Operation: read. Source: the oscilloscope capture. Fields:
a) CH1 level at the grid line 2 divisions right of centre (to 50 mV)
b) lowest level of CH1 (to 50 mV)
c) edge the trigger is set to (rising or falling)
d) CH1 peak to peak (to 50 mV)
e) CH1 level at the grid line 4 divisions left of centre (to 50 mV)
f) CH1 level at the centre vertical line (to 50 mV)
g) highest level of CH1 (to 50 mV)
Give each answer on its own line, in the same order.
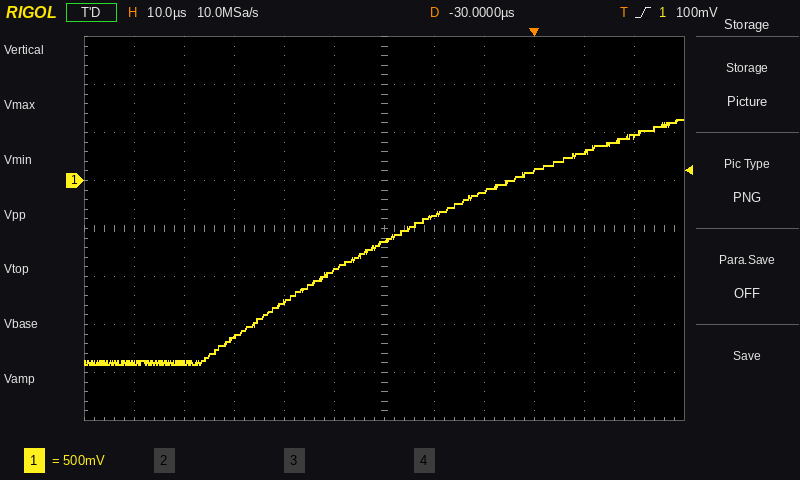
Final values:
-100 mV
-1.90 V
rising
2.55 V
-1.90 V
-600 mV
650 mV
